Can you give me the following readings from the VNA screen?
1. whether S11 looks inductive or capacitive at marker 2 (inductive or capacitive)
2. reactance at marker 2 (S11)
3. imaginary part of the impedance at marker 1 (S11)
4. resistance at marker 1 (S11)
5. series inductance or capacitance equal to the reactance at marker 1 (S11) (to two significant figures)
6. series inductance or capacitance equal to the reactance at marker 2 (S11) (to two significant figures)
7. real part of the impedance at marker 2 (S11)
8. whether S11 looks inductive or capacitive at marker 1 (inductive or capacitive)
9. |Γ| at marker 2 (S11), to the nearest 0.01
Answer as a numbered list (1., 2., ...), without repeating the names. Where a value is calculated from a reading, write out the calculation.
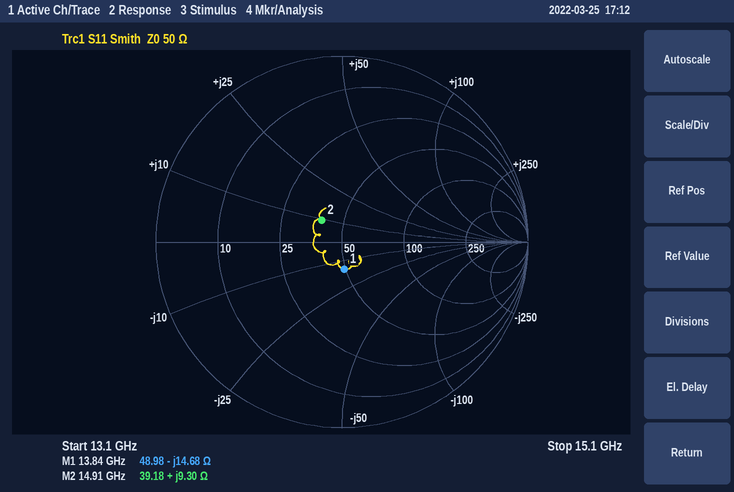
1. inductive
2. +9.30 Ω
3. -14.68 Ω
4. 48.98 Ω
5. C = 1/(2π × 13.84 GHz × 14.68 Ω) ≈ 783 fF, so 780 fF to two significant figures
6. L = 9.3 Ω/(2π × 14.91 GHz) ≈ 99 pH
7. 39.18 Ω
8. capacitive
9. 0.16
